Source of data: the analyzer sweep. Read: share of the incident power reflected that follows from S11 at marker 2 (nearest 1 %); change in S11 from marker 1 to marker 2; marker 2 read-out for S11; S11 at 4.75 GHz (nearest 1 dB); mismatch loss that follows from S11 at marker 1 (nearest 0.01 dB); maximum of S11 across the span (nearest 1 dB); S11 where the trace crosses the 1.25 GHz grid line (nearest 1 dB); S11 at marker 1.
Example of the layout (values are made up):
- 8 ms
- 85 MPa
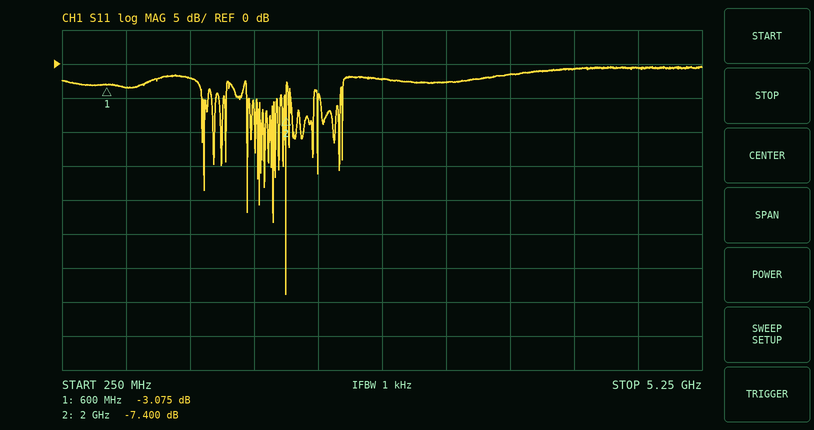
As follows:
- 18 %
- -4.325 dB
- -7.400 dB
- -1 dB
- 2.95 dB
- 0 dB
- -2 dB
- -3.075 dB
